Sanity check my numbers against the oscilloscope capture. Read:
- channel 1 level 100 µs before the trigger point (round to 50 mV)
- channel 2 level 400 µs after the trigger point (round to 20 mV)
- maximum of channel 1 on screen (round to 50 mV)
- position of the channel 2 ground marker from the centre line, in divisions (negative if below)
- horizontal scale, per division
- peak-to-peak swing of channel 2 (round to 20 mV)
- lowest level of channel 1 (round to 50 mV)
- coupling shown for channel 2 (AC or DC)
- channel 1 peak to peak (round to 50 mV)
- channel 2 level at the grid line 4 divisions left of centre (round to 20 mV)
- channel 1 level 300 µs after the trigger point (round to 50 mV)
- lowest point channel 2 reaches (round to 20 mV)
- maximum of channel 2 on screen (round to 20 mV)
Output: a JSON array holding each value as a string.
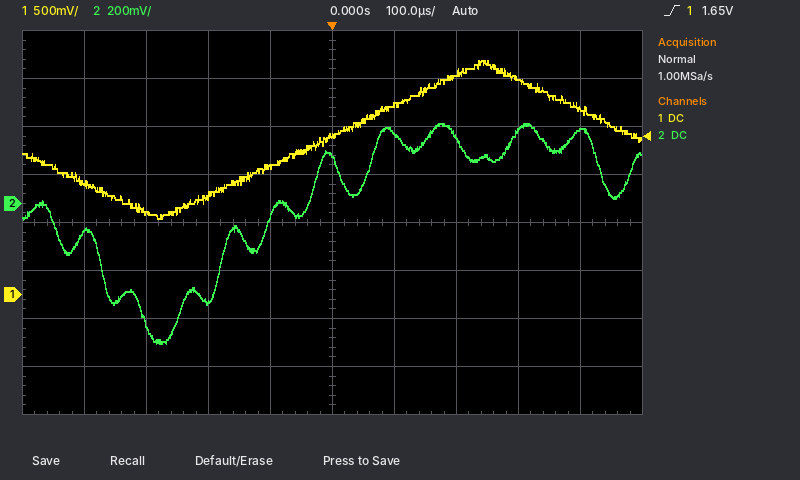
["1.35 V", "300 mV", "2.45 V", "+0.4 div", "100 µs", "920 mV", "800 mV", "DC", "1.65 V", "-120 mV", "2.25 V", "-580 mV", "340 mV"]
